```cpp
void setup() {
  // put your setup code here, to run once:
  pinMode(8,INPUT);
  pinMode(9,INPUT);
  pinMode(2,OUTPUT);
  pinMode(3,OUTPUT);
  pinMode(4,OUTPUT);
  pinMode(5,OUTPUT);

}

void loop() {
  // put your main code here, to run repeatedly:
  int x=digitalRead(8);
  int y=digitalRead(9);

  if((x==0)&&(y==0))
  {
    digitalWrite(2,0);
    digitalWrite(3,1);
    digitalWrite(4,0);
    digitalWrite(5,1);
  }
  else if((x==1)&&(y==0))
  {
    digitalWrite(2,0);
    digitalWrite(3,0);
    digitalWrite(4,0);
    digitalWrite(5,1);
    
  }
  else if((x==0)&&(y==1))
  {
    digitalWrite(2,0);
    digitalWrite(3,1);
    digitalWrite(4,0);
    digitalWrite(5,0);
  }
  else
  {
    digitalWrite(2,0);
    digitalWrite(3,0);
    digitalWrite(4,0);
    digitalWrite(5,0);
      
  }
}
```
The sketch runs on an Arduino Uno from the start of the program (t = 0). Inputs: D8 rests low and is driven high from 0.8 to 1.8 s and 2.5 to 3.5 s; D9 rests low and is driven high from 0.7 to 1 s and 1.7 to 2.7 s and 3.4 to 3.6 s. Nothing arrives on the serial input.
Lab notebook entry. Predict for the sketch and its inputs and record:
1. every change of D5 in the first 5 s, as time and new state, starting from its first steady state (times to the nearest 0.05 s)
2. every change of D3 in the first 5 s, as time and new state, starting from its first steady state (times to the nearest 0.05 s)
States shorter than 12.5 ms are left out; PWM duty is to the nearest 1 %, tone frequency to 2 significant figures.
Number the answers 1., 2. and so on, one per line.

1. 0 s high; 0.7 s low; 1 s high; 1.7 s low; 2.7 s high; 3.4 s low; 3.6 s high
2. 0 s high; 0.8 s low; 1.8 s high; 2.5 s low; 3.5 s high
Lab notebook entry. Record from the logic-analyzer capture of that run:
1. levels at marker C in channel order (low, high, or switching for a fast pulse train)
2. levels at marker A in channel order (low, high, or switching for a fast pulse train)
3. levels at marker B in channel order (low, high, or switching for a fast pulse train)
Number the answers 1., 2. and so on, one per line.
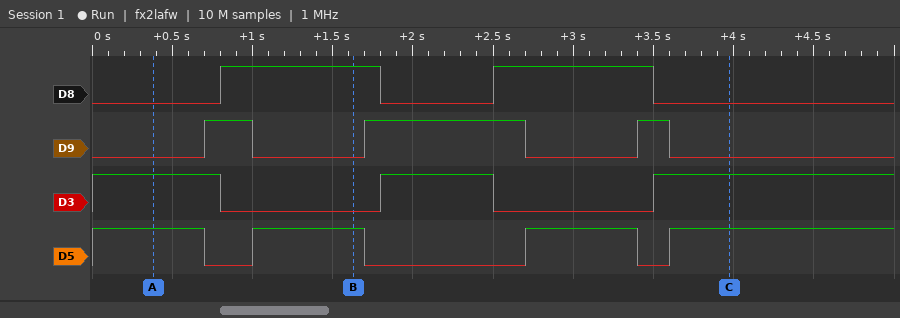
1. D8 low, D9 low, D3 high, D5 high
2. D8 low, D9 low, D3 high, D5 high
3. D8 high, D9 low, D3 low, D5 high
